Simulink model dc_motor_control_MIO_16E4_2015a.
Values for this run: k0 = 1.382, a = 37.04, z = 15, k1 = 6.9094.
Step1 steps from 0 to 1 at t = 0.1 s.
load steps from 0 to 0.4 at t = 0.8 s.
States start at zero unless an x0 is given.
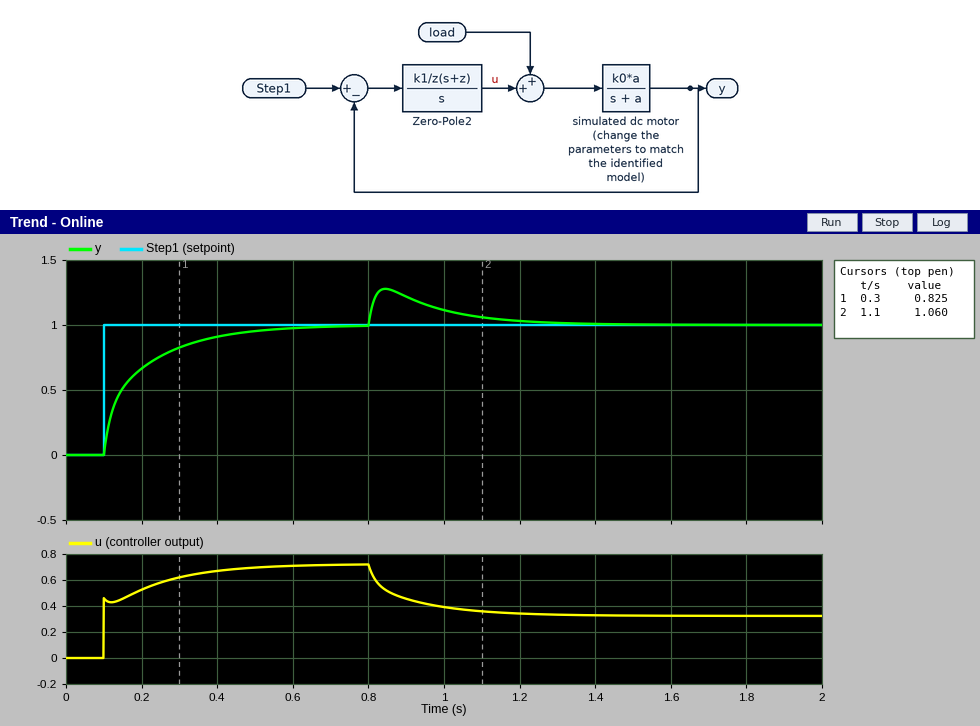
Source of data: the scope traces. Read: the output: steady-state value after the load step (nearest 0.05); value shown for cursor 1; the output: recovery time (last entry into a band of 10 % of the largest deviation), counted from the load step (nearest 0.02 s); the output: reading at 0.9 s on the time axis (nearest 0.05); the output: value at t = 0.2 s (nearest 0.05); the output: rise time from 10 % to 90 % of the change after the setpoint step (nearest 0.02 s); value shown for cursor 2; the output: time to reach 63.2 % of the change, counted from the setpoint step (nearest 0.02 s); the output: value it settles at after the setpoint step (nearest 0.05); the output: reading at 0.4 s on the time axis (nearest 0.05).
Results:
1.00
0.825
0.42 s
1.20
0.65
0.28 s
1.060
0.08 s
1.00
0.90
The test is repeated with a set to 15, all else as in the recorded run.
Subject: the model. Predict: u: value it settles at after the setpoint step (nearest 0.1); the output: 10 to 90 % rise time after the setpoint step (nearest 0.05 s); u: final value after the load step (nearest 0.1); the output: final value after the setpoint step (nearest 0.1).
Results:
0.7
0.25 s
0.3
1.0
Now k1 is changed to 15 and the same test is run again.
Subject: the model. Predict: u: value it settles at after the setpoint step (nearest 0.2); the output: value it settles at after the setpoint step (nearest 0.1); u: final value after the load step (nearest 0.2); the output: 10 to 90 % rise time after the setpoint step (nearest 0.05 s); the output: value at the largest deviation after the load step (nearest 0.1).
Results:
0.8
1.0
0.4
0.15 s
1.2
